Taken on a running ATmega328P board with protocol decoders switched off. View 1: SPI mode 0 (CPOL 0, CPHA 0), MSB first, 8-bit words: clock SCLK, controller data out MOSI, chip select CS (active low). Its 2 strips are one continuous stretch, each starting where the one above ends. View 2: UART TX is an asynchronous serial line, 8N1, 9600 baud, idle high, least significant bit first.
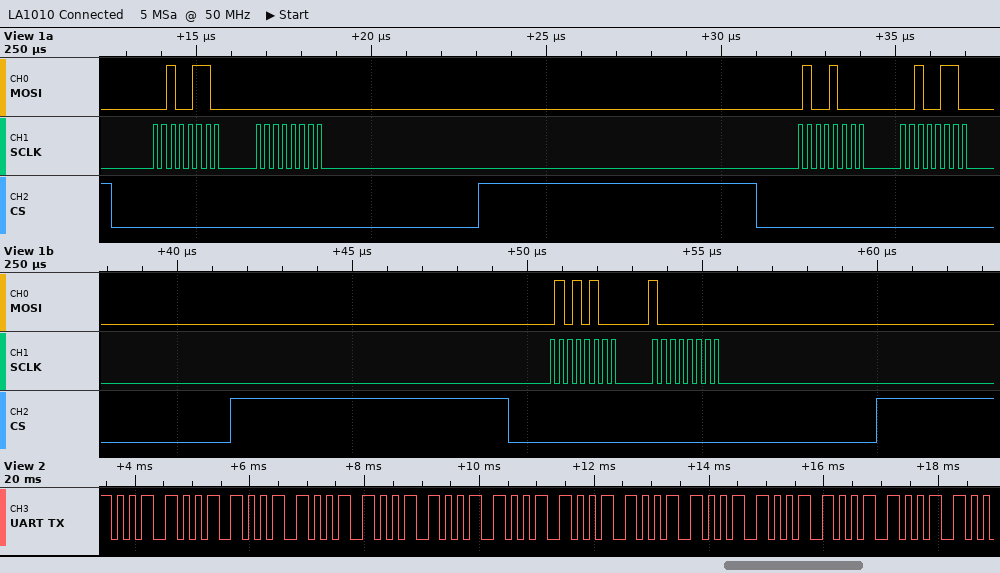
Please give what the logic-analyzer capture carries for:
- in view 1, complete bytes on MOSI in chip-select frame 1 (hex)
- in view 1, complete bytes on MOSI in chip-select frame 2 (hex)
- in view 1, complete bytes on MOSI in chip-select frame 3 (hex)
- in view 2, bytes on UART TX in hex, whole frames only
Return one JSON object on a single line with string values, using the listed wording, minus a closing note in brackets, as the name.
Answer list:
{"in view 1, complete bytes on MOSI in chip-select frame 1": "26 00", "in view 1, complete bytes on MOSI in chip-select frame 2": "48 26", "in view 1, complete bytes on MOSI in chip-select frame 3": "54 80", "in view 2, bytes on UART TX in hex, whole frames only": "0x35 0x35 0x35 0x35 0x35 0x35 0x35 0x35 0x35 0x35 0x35 0x35 0x35"}
